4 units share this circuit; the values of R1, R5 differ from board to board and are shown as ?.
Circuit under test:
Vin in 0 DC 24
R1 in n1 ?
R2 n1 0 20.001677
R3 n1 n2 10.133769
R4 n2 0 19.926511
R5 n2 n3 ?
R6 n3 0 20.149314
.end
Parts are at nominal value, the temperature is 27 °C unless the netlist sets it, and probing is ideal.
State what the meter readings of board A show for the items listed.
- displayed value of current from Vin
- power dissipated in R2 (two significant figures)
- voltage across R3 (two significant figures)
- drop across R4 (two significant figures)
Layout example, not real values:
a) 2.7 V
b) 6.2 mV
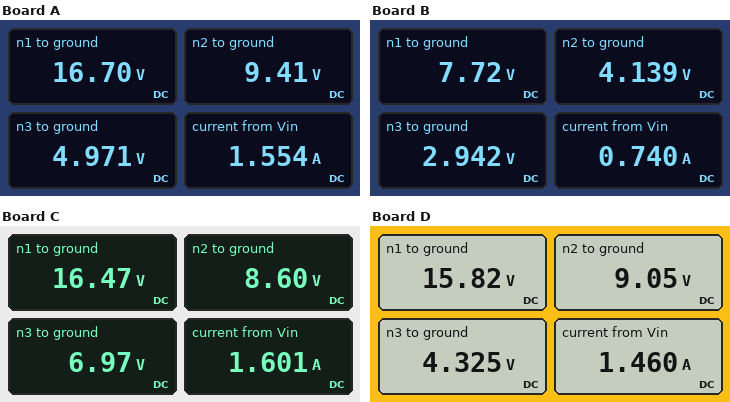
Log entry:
a) 1.554 A
b) 14 W
c) 7.3 V
d) 9.4 V
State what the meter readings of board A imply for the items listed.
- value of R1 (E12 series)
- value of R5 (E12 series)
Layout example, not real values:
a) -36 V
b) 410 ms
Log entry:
a) 4.7 Ω
b) 18 Ω
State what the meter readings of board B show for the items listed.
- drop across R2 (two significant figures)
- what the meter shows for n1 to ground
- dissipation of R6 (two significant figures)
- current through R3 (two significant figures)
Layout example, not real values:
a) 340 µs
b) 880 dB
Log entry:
a) 7.7 V
b) 7.72 V
c) 430 mW
d) 350 mA
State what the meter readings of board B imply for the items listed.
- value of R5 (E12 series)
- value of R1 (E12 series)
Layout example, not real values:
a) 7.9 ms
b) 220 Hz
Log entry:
a) 8.2 Ω
b) 22 Ω
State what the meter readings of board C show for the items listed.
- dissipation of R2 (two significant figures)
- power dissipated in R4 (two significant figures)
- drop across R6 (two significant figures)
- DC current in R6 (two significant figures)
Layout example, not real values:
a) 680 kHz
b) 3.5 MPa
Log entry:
a) 14 W
b) 3.7 W
c) 7.0 V
d) 350 mA
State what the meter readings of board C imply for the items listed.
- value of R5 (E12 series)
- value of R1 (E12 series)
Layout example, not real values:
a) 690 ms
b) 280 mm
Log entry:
a) 4.7 Ω
b) 4.7 Ω
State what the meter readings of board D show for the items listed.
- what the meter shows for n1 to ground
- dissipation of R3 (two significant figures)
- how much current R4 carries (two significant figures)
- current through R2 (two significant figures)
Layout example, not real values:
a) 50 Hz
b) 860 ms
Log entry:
a) 15.82 V
b) 4.5 W
c) 450 mA
d) 790 mA
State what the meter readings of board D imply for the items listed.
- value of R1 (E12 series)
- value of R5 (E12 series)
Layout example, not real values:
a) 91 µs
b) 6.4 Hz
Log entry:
a) 5.6 Ω
b) 22 Ω
